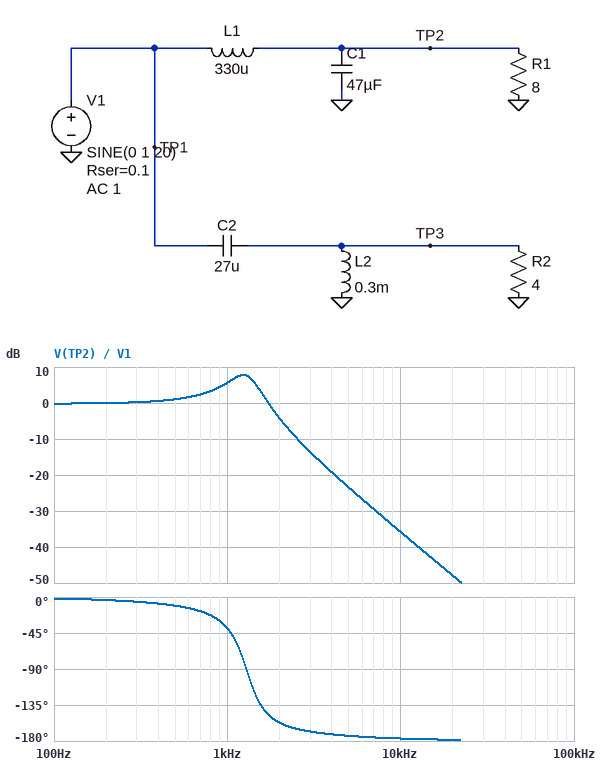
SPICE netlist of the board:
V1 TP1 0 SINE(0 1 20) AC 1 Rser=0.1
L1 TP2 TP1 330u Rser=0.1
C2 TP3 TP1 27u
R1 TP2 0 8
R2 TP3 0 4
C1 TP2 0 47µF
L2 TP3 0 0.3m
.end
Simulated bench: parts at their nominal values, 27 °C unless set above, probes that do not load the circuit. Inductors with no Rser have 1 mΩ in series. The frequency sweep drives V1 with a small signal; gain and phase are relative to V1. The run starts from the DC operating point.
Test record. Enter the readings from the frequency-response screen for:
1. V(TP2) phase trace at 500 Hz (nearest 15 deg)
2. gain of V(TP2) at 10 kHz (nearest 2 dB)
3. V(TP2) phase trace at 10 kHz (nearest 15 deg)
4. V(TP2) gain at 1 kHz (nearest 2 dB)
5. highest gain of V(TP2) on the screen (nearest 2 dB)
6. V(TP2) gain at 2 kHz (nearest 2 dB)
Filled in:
-15 deg
-36 dB
-180 deg
6 dB
8 dB
-4 dB
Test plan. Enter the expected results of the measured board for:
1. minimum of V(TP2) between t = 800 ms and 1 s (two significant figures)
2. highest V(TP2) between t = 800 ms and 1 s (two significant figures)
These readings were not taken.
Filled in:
-980 mV
980 mV
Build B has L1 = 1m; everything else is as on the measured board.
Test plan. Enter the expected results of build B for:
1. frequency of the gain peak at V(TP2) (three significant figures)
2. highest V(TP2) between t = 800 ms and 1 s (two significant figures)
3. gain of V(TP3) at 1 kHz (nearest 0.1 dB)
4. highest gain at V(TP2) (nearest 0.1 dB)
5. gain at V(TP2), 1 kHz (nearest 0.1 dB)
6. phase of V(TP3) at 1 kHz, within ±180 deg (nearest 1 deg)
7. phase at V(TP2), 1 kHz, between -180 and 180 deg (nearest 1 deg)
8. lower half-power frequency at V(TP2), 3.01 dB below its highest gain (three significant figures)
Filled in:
670 Hz
980 mV
-8.4 dB
4.5 dB
-1.5 dB
145 deg
-136 deg
356 Hz
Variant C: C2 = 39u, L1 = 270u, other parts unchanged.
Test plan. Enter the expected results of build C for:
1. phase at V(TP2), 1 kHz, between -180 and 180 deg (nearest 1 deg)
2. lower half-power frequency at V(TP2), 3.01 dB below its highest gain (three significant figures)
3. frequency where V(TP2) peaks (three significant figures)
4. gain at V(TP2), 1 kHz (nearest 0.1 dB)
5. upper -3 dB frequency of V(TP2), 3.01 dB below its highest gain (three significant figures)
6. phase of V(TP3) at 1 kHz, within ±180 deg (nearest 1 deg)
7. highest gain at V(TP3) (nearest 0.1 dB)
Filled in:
-29 deg
1.05 kHz
1.37 kHz
4.5 dB
1.62 kHz
135 deg
2.9 dB
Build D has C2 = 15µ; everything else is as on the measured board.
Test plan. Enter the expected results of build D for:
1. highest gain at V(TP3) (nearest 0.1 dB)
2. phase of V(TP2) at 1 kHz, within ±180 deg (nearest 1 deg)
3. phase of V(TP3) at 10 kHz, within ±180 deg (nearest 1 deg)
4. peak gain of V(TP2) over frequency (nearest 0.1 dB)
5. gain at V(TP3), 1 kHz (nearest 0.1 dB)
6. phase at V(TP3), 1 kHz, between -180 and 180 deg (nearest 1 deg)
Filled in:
0.4 dB
-38 deg
16 deg
7.9 dB
-15.0 dB
148 deg
